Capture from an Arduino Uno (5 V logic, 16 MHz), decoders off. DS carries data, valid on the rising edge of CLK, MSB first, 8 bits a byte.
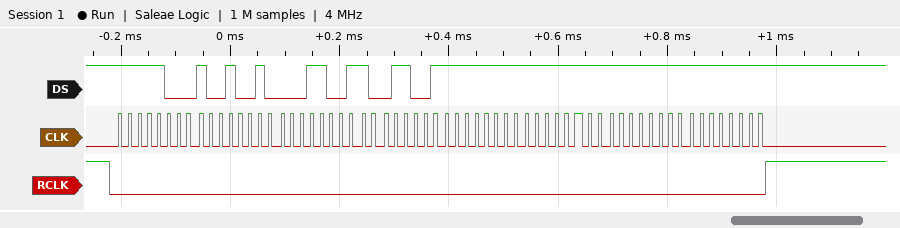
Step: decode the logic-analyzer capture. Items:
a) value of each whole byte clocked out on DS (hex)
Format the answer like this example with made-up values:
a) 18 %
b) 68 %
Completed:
a) F8 92 19 99 FF FF FF FF
